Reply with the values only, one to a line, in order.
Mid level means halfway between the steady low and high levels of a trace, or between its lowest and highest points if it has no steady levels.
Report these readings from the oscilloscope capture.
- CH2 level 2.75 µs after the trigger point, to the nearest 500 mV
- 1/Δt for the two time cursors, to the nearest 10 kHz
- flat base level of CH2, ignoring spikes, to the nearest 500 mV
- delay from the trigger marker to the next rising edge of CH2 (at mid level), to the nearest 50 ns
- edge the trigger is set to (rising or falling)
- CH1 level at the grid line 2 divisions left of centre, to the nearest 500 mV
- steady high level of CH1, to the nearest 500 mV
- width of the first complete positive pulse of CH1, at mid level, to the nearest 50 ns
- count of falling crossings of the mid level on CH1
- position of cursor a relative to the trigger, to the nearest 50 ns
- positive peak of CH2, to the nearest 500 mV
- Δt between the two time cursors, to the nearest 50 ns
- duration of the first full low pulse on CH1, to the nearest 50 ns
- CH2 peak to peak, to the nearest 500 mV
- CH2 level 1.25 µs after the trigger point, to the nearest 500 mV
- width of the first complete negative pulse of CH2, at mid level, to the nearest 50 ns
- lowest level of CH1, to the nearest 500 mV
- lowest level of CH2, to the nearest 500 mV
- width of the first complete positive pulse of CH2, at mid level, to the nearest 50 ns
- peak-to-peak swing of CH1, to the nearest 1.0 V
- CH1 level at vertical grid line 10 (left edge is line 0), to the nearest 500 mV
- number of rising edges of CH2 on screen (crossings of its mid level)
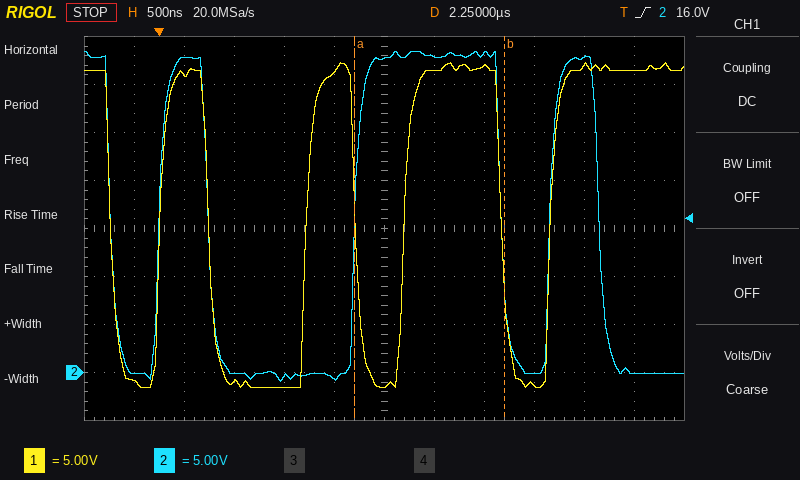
33.0 V
670 kHz
0.0 V
1.95 µs
rising
-1.5 V
31.5 V
500 ns
4
+1.95 µs
33.5 V
1.50 µs
500 ns
34.5 V
-500 mV
500 ns
-1.5 V
-1.0 V
500 ns
34.0 V
32.0 V
3
